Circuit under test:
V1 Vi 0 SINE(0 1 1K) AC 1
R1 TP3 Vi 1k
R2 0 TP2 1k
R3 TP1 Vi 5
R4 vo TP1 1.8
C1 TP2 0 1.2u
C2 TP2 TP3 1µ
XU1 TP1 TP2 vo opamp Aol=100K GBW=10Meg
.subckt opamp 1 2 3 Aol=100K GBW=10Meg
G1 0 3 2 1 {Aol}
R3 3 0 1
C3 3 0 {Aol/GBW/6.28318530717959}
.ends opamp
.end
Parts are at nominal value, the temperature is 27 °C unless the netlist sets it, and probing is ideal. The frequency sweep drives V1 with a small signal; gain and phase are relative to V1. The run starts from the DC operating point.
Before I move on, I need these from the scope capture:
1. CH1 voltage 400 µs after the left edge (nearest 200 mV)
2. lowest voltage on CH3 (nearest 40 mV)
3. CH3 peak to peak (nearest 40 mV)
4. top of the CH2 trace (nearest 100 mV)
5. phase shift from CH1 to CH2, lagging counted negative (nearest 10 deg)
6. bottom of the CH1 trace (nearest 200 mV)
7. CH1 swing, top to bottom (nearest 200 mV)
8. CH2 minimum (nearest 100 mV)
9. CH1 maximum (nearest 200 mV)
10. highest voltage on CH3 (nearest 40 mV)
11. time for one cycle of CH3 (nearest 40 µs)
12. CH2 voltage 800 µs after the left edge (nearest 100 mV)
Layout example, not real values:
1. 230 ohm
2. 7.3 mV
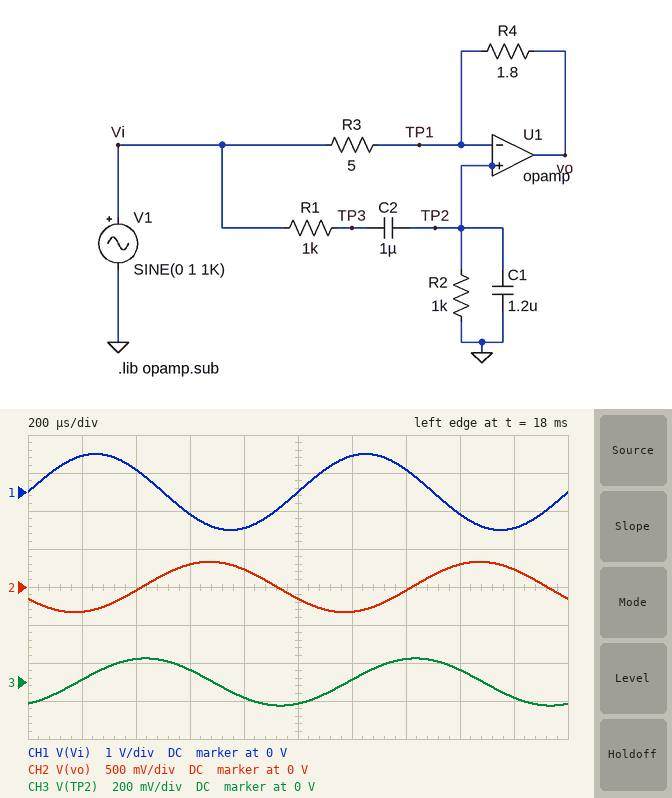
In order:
1. 600 mV
2. -120 mV
3. 240 mV
4. 300 mV
5. -150 deg
6. -1.0 V
7. 2.0 V
8. -300 mV
9. 1.0 V
10. 120 mV
11. 1.00 ms
12. 200 mV
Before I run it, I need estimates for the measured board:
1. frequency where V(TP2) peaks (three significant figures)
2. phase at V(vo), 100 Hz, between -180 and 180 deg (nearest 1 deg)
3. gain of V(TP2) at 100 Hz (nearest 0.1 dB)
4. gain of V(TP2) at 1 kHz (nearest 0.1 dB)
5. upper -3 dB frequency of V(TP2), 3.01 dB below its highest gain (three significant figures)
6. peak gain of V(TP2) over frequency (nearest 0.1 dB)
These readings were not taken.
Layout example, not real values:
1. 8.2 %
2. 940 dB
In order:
1. 145 Hz
2. 70 deg
3. -10.4 dB
4. -18.1 dB
5. 469 Hz
6. -10.1 dB
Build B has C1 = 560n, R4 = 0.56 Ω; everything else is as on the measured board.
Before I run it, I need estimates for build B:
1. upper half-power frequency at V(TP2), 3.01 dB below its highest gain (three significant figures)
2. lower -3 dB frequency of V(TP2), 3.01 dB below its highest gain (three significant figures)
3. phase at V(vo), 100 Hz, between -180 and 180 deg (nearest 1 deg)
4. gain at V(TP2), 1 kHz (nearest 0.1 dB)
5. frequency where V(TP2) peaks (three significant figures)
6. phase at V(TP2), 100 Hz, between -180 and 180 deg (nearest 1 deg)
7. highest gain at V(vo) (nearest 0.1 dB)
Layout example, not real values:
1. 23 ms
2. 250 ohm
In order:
1. 785 Hz
2. 57.6 Hz
3. 35 deg
4. -12.5 dB
5. 213 Hz
6. 26 deg
7. -9.8 dB
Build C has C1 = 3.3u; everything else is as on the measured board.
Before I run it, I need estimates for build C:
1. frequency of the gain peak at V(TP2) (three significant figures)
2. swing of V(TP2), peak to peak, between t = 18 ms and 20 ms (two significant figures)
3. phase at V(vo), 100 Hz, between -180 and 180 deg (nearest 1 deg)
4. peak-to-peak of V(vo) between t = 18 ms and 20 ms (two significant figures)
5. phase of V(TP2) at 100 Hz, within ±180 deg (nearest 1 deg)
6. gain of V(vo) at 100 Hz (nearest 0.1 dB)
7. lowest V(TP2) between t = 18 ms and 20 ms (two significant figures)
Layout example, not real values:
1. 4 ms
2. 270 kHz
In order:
1. 87.6 Hz
2. 94 mV
3. -168 deg
4. 700 mV
5. -5 deg
6. -19.3 dB
7. -47 mV
